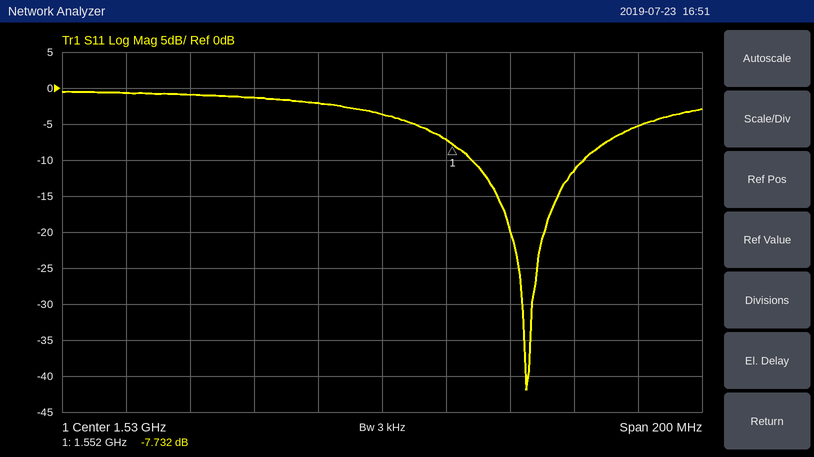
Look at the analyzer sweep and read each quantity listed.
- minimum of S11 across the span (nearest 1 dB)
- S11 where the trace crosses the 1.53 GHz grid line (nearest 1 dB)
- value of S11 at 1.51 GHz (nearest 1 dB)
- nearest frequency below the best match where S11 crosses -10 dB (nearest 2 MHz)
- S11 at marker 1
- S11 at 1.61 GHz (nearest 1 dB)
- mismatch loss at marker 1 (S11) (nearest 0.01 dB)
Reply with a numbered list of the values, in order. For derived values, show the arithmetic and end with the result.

1. -42 dB
2. -4 dB
3. -2 dB
4. 1.558 GHz
5. -7.732 dB
6. -5 dB
7. −10 log10(1 − 10^(-7.732/10)) ≈ 0.80 dB
